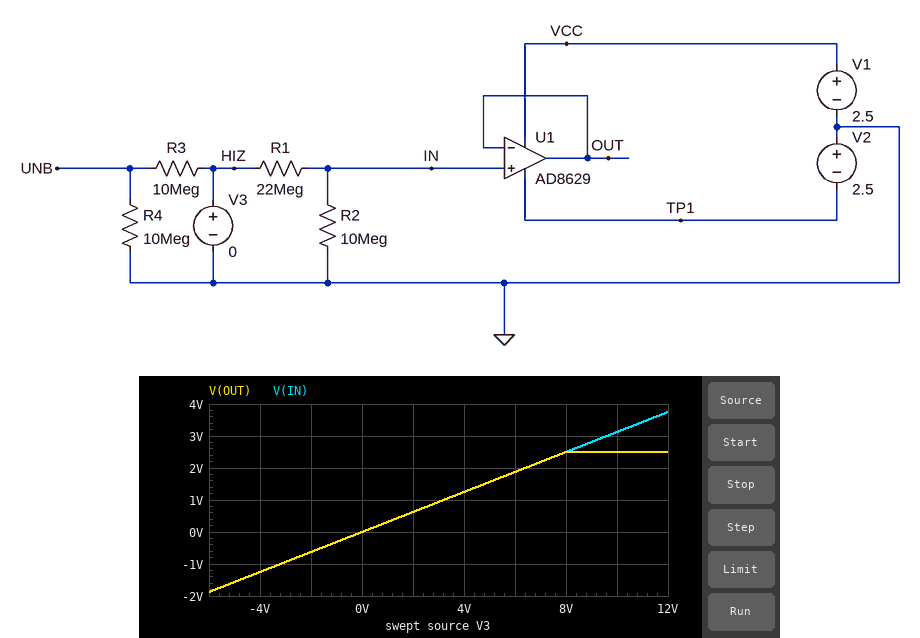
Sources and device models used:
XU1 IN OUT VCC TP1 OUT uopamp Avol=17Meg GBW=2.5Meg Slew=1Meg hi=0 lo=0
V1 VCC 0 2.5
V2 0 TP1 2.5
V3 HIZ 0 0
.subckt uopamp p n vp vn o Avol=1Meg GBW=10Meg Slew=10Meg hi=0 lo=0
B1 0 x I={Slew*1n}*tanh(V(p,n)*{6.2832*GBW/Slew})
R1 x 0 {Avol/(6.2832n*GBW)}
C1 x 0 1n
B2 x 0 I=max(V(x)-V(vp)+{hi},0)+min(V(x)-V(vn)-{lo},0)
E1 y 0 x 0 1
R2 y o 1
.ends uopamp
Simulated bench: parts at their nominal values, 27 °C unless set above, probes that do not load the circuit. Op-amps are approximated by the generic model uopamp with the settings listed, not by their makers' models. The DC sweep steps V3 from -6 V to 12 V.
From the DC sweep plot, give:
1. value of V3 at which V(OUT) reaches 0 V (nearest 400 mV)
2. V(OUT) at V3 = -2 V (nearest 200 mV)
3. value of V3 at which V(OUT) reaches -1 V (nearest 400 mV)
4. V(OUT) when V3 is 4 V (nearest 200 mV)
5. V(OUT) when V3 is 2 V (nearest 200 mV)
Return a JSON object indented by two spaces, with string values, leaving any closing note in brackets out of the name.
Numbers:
{
  "value of V3 at which V(OUT) reaches 0 V": "0 V",
  "V(OUT) at V3 = -2 V": "-600 mV",
  "value of V3 at which V(OUT) reaches -1 V": "-3.2 V",
  "V(OUT) when V3 is 4 V": "1.2 V",
  "V(OUT) when V3 is 2 V": "600 mV"
}
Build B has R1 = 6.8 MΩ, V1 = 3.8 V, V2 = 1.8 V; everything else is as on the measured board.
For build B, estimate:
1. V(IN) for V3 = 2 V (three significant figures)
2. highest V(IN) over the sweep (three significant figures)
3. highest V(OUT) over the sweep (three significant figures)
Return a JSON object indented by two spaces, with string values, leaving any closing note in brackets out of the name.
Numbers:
{
  "V(IN) for V3 = 2 V": "1.19 V",
  "highest V(IN) over the sweep": "7.14 V",
  "highest V(OUT) over the sweep": "3.80 V"
}
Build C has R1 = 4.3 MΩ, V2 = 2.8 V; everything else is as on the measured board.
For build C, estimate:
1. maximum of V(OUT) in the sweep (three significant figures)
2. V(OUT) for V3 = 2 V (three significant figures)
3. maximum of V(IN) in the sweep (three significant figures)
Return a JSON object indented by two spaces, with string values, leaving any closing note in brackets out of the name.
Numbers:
{
  "maximum of V(OUT) in the sweep": "2.50 V",
  "V(OUT) for V3 = 2 V": "1.40 V",
  "maximum of V(IN) in the sweep": "8.39 V"
}
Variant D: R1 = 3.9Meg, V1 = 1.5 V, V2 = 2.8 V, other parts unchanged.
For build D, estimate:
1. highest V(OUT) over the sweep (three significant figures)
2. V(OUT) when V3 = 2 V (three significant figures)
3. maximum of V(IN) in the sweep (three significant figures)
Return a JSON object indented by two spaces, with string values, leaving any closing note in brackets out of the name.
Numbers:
{
  "highest V(OUT) over the sweep": "1.50 V",
  "V(OUT) when V3 = 2 V": "1.44 V",
  "maximum of V(IN) in the sweep": "8.63 V"
}
